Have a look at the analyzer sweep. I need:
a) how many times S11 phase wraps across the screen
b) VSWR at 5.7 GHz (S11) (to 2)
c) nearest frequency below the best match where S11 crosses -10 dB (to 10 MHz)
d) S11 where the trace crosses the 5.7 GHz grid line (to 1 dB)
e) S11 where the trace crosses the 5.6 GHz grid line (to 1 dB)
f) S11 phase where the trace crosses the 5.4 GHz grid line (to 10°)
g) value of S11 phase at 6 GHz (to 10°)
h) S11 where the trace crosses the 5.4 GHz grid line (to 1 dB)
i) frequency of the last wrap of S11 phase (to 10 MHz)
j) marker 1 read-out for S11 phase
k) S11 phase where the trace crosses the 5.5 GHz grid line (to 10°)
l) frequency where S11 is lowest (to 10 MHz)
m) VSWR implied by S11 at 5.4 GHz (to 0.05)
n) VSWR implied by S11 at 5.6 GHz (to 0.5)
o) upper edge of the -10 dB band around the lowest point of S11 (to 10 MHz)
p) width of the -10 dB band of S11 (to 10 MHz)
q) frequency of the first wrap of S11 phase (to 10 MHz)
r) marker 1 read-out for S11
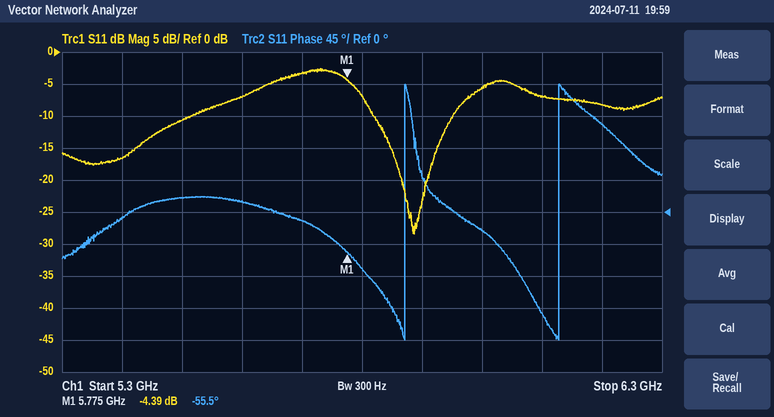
2
6
5.82 GHz
-3 dB
-7 dB
-10°
-30°
-17 dB
6.13 GHz
-55.5°
20°
5.89 GHz
1.35
2.5
5.95 GHz
130 MHz
5.87 GHz
-4.39 dB
